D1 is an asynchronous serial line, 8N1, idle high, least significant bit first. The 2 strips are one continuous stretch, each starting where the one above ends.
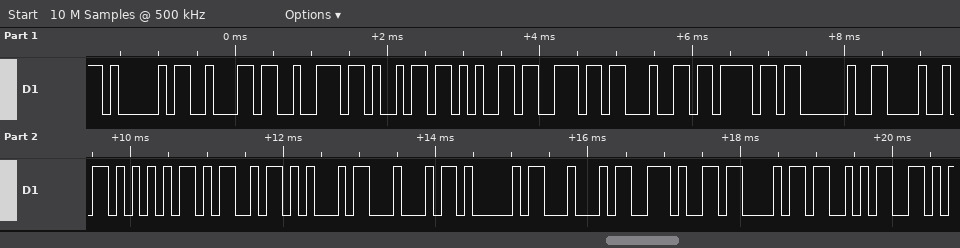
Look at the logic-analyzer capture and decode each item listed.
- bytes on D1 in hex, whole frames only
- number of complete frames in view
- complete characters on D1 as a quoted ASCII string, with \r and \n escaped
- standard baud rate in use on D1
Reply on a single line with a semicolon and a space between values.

0x41 0x62 0x72 0x69 0x65 0x6E 0x64 0x6F 0x20 0x48 0x55 0x4D 0x45 0x44 0x41 0x44 0x2E 0x43 0x53; 19; "Abriendo HUMEDAD.CS"; 9600 baud
